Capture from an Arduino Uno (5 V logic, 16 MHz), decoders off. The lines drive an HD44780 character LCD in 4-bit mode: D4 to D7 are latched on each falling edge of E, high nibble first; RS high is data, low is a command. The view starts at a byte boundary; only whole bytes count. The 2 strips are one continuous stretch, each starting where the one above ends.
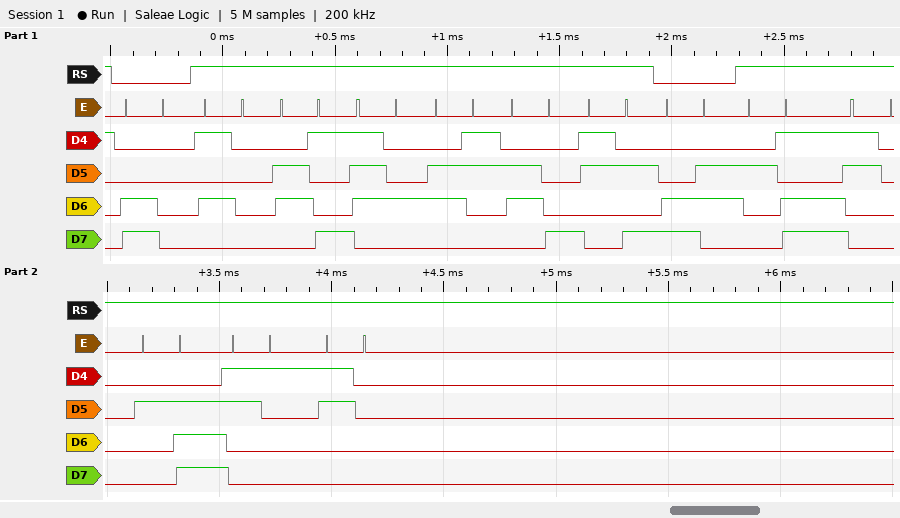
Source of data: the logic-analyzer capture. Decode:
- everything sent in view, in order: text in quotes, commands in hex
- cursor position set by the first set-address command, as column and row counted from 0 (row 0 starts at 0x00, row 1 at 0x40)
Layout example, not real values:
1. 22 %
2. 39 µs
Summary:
1. 0xC0 "Pitch:" 0xC6 "-0.10"
2. column 0, row 1
